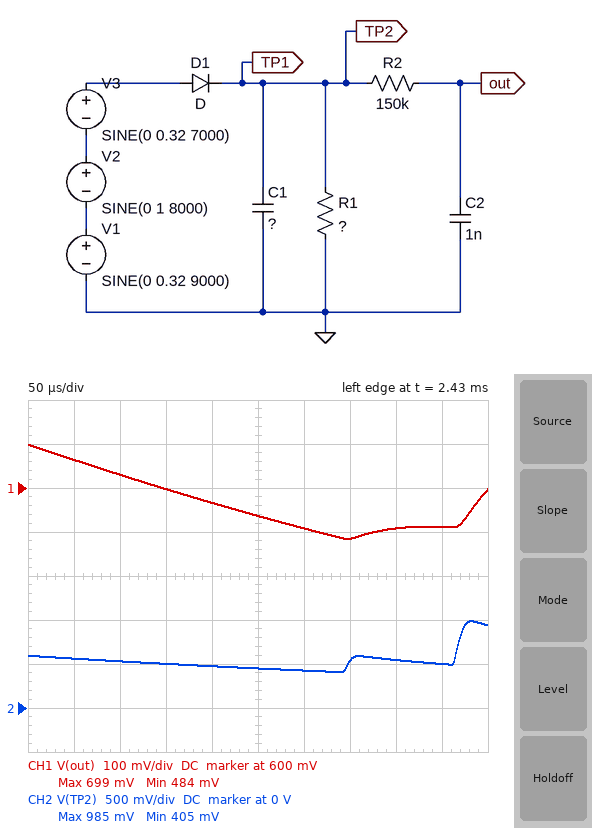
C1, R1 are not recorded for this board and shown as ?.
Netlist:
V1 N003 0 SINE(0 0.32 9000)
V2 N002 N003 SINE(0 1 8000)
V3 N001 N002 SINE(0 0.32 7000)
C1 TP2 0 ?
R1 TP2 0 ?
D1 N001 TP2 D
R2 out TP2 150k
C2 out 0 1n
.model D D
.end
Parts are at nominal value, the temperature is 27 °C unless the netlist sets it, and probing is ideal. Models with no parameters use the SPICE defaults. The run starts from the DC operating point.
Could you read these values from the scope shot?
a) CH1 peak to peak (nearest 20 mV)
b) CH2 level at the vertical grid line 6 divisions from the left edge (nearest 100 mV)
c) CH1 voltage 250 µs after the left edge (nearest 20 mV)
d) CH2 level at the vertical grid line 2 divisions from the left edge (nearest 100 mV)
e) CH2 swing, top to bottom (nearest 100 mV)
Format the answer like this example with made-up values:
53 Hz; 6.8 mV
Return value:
220 mV; 400 mV; 540 mV; 500 mV; 600 mV
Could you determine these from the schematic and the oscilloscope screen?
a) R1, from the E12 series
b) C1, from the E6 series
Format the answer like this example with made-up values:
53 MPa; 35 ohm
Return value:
270 kΩ; 2.2 nF
